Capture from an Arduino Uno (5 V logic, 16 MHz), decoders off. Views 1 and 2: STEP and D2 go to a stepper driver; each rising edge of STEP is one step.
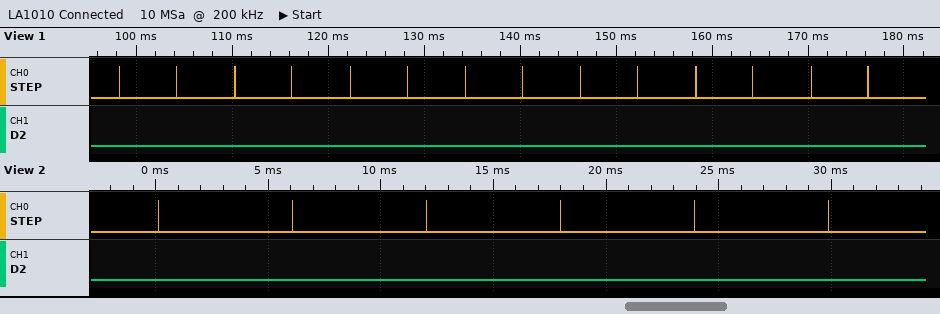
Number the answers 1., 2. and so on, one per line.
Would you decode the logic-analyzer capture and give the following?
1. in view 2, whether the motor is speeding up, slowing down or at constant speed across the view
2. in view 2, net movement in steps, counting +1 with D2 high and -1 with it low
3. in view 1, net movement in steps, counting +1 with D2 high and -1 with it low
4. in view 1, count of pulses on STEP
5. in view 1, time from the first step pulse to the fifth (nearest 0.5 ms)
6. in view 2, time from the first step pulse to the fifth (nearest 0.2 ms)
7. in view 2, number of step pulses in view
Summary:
1. constant speed
2. -6
3. -14
4. 14
5. 24.0 ms
6. 23.8 ms
7. 6
